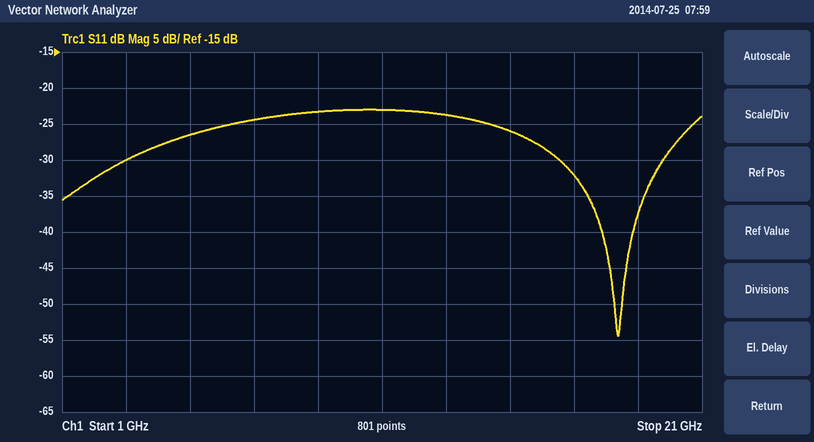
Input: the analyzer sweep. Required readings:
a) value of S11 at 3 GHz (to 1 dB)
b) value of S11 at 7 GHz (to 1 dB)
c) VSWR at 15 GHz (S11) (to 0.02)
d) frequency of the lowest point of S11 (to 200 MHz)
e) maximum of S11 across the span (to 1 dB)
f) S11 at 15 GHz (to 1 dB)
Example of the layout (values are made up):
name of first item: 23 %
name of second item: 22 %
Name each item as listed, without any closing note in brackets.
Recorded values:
value of S11 at 3 GHz: -30 dB
value of S11 at 7 GHz: -24 dB
VSWR at 15 GHz (S11): 1.10
frequency of the lowest point of S11: 18.4 GHz
maximum of S11 across the span: -23 dB
S11 at 15 GHz: -26 dB
